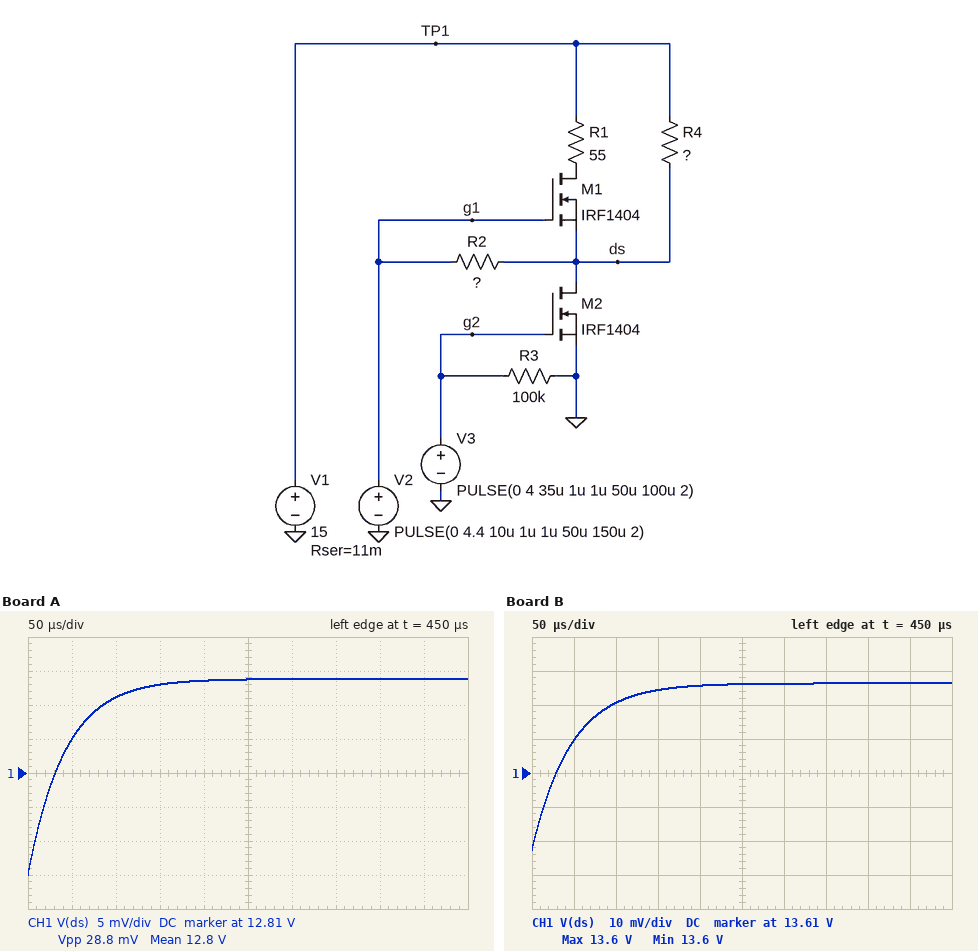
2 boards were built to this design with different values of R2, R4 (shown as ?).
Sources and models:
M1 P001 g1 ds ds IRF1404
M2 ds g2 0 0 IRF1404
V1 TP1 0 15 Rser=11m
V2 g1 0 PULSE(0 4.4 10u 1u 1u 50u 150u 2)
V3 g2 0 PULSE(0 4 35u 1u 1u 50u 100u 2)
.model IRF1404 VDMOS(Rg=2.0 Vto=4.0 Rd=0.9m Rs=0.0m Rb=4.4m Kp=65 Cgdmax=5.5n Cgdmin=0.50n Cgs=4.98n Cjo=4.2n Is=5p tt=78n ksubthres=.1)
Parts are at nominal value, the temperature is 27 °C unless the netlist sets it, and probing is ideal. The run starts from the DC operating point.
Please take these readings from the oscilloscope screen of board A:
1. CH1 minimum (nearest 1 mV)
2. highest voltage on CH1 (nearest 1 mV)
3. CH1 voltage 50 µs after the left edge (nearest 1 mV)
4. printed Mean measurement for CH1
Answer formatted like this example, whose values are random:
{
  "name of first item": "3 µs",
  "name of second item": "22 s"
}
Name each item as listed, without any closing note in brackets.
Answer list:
{
  "CH1 minimum": "12.795 V",
  "highest voltage on CH1": "12.824 V",
  "CH1 voltage 50 µs after the left edge": "12.815 V",
  "printed Mean measurement for CH1": "12.8 V"
}
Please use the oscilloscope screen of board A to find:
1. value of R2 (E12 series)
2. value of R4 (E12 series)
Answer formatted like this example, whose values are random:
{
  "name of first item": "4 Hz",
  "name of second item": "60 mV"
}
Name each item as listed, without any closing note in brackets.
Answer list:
{
  "value of R2": "33 kΩ",
  "value of R4": "5.6 kΩ"
}
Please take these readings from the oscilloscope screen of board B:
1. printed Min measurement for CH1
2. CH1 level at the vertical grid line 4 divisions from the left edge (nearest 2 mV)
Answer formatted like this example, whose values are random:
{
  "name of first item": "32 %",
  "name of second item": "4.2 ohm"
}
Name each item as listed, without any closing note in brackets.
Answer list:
{
  "printed Min measurement for CH1": "13.6 V",
  "CH1 level at the vertical grid line 4 divisions from the left edge": "13.636 V"
}
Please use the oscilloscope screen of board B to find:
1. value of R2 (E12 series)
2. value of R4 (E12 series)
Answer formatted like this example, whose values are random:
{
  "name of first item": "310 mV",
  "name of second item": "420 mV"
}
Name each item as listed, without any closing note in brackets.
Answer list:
{
  "value of R2": "56 kΩ",
  "value of R4": "5.6 kΩ"
}
